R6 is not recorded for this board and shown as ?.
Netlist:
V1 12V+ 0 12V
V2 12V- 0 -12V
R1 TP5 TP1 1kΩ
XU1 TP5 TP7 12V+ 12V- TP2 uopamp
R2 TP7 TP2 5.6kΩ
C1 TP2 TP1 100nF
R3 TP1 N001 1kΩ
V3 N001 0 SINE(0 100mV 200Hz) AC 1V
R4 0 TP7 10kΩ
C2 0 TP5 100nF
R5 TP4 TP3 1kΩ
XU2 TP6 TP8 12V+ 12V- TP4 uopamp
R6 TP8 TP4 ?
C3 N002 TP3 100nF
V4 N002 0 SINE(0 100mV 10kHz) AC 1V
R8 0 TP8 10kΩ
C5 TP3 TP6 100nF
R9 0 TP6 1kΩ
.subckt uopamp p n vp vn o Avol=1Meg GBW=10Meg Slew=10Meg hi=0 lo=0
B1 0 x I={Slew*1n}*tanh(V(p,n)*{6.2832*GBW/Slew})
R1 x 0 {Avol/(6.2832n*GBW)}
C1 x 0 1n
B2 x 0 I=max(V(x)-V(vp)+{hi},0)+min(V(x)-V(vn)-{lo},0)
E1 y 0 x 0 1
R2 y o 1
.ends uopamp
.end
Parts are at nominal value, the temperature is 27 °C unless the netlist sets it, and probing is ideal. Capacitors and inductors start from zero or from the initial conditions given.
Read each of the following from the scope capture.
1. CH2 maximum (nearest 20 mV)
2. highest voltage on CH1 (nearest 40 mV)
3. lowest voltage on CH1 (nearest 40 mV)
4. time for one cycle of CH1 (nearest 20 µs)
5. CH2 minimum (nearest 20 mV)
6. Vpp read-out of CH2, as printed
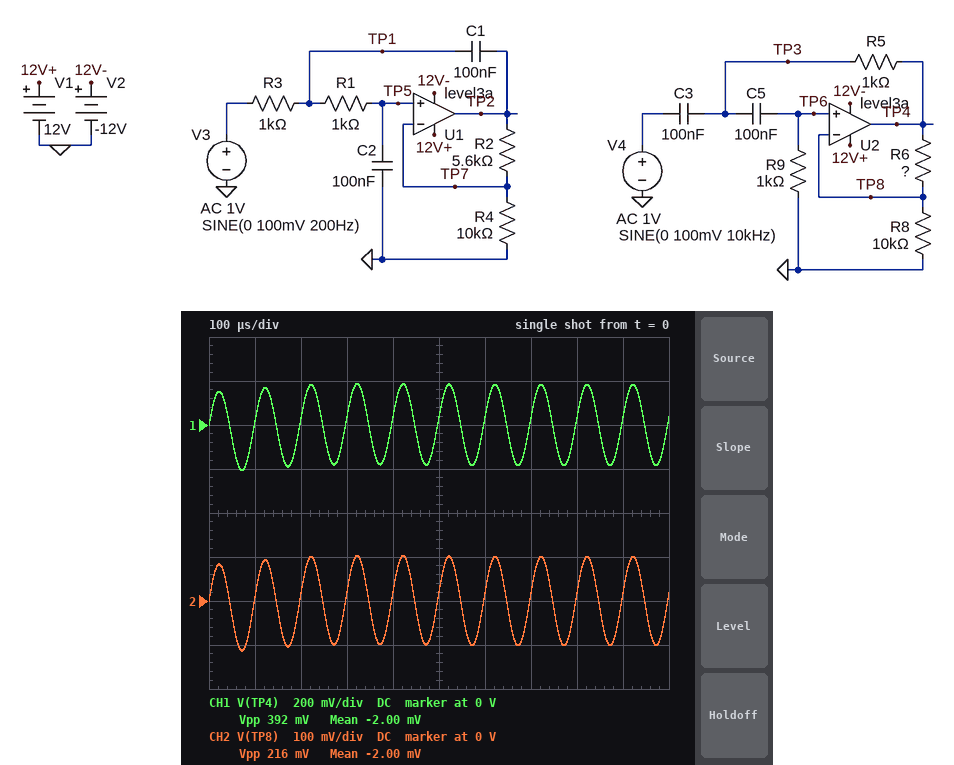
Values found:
100 mV
200 mV
-200 mV
100 µs
-120 mV
216 mV
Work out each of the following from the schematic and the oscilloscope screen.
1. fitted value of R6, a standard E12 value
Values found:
8.2 kΩ
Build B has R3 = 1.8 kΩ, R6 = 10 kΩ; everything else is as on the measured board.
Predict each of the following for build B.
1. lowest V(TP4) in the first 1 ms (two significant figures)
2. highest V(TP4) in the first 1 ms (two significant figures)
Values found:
-230 mV
210 mV
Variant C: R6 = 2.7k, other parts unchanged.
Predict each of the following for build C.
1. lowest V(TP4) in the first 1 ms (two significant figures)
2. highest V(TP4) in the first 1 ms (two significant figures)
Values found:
-140 mV
130 mV
